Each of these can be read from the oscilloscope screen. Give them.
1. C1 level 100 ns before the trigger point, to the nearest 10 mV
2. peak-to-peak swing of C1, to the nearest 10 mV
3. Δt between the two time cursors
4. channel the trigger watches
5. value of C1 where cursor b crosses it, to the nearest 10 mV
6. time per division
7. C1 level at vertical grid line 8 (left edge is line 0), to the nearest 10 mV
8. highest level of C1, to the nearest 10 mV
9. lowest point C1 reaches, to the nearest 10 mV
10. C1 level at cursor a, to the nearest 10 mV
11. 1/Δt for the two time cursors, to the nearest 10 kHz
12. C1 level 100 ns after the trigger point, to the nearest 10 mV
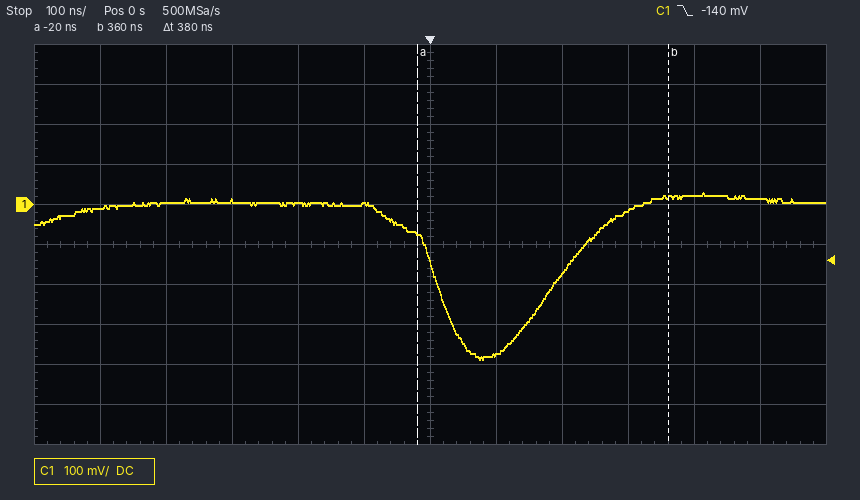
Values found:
0 mV
420 mV
380 ns
C1
20 mV
100 ns
-170 mV
30 mV
-390 mV
-70 mV
2.63 MHz
-380 mV
